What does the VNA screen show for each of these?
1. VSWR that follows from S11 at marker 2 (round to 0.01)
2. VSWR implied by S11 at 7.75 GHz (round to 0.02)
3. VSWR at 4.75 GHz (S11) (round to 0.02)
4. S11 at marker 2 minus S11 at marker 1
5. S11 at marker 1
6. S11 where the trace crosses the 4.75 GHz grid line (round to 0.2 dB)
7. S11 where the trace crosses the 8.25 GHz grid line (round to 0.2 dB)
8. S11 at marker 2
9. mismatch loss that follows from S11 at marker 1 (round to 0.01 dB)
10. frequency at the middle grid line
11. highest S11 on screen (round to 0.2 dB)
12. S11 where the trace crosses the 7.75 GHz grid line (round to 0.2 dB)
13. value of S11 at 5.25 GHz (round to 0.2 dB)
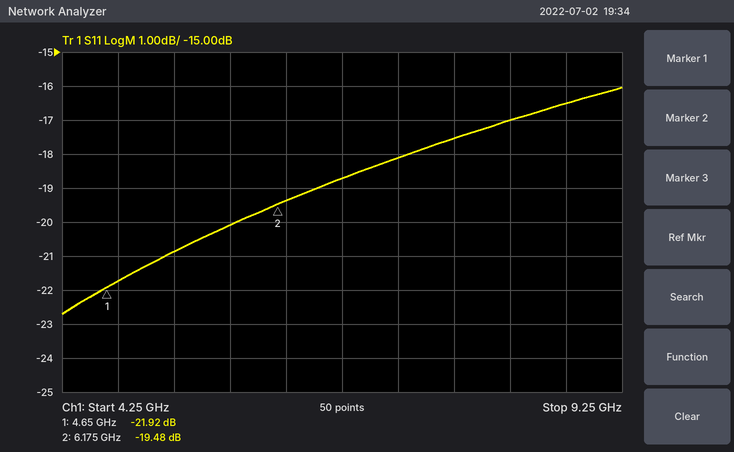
1.24
1.30
1.18
2.44 dB
-21.92 dB
-21.8 dB
-17.0 dB
-19.48 dB
0.03 dB
6.75 GHz
-16.0 dB
-17.6 dB
-20.8 dB
